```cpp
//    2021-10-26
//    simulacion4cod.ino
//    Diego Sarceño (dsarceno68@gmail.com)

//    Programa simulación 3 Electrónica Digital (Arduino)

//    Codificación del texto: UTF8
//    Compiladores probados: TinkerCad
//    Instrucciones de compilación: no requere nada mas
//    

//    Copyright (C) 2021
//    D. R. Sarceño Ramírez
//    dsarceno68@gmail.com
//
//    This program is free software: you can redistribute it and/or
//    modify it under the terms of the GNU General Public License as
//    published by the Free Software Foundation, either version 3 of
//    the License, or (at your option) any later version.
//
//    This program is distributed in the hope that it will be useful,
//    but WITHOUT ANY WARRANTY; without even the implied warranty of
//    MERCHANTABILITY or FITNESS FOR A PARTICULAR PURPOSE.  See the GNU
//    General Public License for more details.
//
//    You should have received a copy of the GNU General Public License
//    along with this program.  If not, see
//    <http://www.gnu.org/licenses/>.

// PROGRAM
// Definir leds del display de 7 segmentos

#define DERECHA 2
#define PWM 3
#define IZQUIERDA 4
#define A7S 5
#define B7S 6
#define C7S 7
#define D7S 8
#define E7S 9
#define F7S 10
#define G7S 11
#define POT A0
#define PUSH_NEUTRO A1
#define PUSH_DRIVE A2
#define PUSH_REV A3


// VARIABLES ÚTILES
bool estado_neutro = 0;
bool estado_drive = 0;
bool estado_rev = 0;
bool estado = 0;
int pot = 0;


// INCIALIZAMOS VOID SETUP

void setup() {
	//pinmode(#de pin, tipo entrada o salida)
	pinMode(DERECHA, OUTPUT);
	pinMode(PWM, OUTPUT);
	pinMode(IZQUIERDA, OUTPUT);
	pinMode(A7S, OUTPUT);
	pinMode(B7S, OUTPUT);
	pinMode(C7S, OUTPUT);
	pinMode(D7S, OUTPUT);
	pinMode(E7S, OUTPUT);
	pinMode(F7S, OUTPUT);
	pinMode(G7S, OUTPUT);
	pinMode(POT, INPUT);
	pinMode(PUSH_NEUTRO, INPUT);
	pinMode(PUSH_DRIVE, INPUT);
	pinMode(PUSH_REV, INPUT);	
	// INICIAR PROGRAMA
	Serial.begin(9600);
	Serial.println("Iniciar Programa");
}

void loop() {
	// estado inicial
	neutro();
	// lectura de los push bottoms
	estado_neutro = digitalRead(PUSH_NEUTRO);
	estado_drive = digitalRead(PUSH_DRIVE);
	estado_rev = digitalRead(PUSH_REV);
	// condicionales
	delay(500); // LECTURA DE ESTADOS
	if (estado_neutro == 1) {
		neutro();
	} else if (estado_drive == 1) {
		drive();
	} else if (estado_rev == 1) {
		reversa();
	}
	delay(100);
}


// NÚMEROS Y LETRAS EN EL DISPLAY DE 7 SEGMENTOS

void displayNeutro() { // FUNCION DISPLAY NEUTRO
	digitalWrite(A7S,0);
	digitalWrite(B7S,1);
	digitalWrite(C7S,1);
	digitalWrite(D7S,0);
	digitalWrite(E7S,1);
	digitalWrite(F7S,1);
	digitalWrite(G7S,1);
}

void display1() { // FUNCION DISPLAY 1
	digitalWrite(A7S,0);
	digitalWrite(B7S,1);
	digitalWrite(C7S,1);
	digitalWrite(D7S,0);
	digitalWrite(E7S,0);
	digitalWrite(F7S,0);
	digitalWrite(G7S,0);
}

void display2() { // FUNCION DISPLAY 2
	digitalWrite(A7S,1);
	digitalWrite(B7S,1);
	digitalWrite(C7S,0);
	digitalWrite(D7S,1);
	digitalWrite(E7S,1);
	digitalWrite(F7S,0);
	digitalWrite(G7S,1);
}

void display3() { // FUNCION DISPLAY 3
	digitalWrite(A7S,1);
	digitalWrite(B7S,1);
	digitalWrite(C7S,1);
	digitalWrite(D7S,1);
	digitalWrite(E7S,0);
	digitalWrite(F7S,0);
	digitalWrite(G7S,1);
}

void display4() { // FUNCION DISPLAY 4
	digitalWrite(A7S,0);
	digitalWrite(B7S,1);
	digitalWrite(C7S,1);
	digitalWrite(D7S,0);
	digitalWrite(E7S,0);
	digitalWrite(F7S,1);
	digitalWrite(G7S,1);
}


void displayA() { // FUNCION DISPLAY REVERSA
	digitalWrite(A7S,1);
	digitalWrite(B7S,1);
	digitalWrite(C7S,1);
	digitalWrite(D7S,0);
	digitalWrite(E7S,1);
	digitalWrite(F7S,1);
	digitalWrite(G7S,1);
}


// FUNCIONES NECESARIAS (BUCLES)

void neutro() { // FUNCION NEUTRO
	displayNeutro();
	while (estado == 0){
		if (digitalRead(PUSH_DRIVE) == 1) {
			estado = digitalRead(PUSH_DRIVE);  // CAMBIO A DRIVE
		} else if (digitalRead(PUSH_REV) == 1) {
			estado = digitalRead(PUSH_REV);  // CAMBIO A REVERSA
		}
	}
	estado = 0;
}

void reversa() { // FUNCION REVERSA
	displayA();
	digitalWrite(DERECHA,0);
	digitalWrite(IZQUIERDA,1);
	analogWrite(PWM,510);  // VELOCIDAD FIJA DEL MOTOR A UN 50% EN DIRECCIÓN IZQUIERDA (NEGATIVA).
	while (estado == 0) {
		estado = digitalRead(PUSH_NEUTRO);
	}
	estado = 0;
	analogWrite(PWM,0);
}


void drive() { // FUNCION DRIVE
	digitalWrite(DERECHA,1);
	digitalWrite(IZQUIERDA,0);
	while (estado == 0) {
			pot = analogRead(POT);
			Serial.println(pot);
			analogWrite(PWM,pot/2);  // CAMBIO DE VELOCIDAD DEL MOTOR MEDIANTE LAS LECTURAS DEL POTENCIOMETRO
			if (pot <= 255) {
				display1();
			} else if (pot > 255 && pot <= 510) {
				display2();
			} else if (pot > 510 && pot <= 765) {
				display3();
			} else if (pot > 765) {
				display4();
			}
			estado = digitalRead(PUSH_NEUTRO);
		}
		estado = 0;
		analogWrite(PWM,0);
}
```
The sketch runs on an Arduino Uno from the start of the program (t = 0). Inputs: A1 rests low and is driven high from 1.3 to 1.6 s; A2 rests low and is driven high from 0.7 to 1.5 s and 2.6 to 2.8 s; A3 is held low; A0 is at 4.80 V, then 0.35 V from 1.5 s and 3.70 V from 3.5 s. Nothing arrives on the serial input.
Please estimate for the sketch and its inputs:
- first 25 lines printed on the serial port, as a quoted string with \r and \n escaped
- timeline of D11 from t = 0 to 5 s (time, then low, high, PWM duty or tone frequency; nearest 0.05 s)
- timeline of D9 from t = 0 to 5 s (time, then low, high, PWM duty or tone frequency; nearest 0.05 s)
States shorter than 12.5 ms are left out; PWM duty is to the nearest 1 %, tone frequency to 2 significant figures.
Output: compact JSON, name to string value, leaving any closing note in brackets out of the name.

{"first 25 lines printed on the serial port, as a quoted string with \\r and \\n escaped": "\"Iniciar Programa\\r\\n983\\r\\n983\\r\\n983\\r\\n983\\r\\n983\\r\\n983\\r\\n983\\r\\n983\\r\\n983\\r\\n983\\r\\n983\\r\\n983\\r\\n983\\r\\n983\\r\\n983\\r\\n983\\r\\n983\\r\\n983\\r\\n983\\r\\n983\\r\\n983\\r\\n983\\r\\n983\\r\\n983\\r\\n\"", "timeline of D11 from t = 0 to 5 s": "0 s high; 3.2 s low; 3.5 s high", "timeline of D9 from t = 0 to 5 s": "0 s high; 1.2 s low; 1.4 s high; 3.2 s low"}
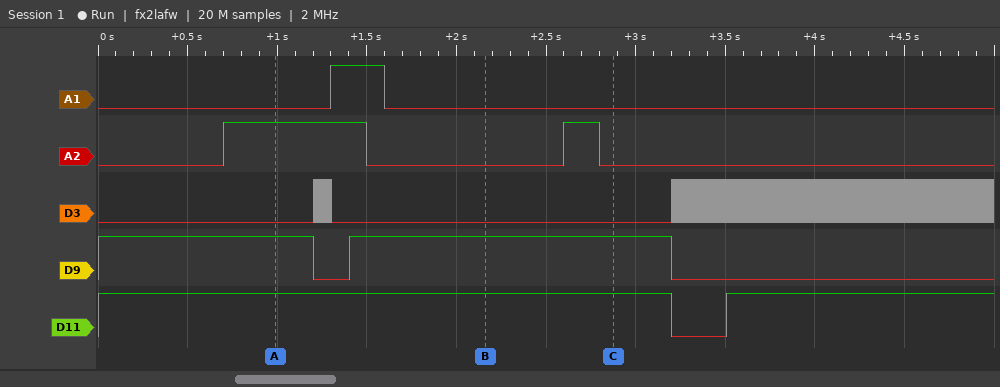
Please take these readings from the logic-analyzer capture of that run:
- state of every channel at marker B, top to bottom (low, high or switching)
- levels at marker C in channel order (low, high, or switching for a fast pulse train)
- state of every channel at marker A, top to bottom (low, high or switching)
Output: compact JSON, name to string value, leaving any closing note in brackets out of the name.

{"state of every channel at marker B, top to bottom": "A1 low, A2 low, D3 low, D9 high, D11 high", "levels at marker C in channel order": "A1 low, A2 low, D3 low, D9 high, D11 high", "state of every channel at marker A, top to bottom": "A1 low, A2 high, D3 low, D9 high, D11 high"}
